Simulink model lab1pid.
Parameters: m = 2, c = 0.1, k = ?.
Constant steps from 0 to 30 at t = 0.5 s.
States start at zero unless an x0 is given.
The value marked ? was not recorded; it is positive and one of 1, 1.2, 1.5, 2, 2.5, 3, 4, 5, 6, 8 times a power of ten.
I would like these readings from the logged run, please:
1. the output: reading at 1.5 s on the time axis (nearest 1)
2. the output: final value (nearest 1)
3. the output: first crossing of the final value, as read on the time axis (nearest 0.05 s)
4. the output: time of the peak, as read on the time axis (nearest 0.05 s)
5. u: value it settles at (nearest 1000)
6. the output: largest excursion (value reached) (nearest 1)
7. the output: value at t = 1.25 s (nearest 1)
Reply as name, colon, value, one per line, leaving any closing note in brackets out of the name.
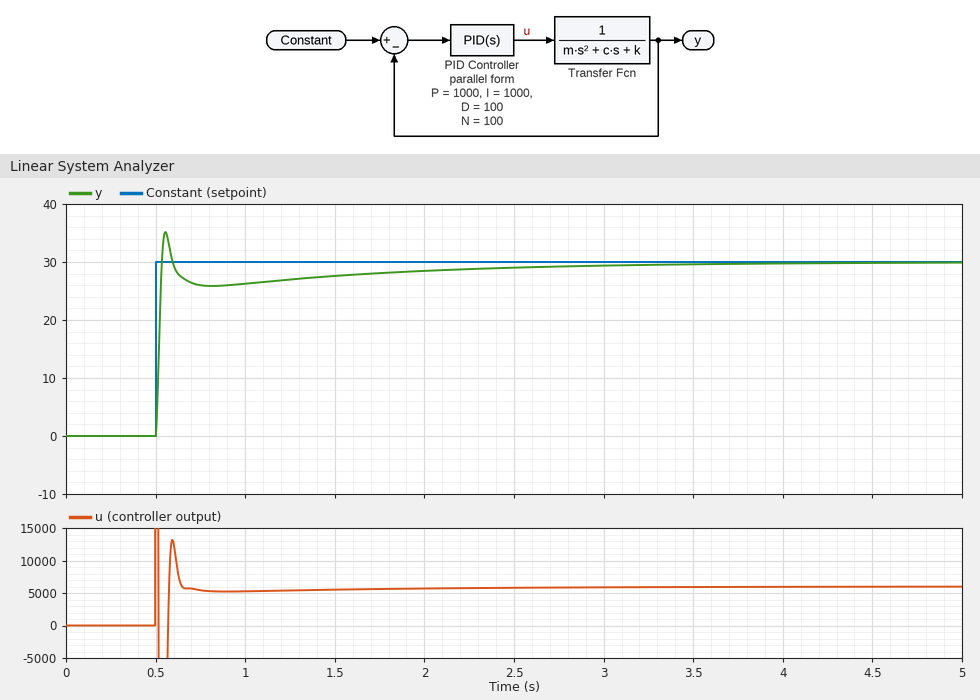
the output: reading at 1.5 s on the time axis: 28
the output: final value: 30
the output: first crossing of the final value, as read on the time axis: 0.55 s
the output: time of the peak, as read on the time axis: 0.55 s
u: value it settles at: 6000
the output: largest excursion (value reached): 35
the output: value at t = 1.25 s: 27
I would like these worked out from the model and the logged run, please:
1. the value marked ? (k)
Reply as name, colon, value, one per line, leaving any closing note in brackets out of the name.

the value marked ?: 200
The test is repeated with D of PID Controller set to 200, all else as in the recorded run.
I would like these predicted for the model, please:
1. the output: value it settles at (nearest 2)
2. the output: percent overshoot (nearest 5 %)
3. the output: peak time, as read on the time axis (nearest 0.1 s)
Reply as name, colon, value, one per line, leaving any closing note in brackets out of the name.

the output: value it settles at: 30
the output: percent overshoot: 20 %
the output: peak time, as read on the time axis: 0.5 s
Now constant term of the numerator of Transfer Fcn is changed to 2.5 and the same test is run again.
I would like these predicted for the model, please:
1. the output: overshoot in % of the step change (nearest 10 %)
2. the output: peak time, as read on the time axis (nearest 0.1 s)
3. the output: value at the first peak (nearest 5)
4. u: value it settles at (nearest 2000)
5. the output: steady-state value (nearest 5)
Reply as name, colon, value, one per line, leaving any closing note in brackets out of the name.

the output: overshoot in % of the step change: 30 %
the output: peak time, as read on the time axis: 0.5 s
the output: value at the first peak: 40
u: value it settles at: 2000
the output: steady-state value: 30
